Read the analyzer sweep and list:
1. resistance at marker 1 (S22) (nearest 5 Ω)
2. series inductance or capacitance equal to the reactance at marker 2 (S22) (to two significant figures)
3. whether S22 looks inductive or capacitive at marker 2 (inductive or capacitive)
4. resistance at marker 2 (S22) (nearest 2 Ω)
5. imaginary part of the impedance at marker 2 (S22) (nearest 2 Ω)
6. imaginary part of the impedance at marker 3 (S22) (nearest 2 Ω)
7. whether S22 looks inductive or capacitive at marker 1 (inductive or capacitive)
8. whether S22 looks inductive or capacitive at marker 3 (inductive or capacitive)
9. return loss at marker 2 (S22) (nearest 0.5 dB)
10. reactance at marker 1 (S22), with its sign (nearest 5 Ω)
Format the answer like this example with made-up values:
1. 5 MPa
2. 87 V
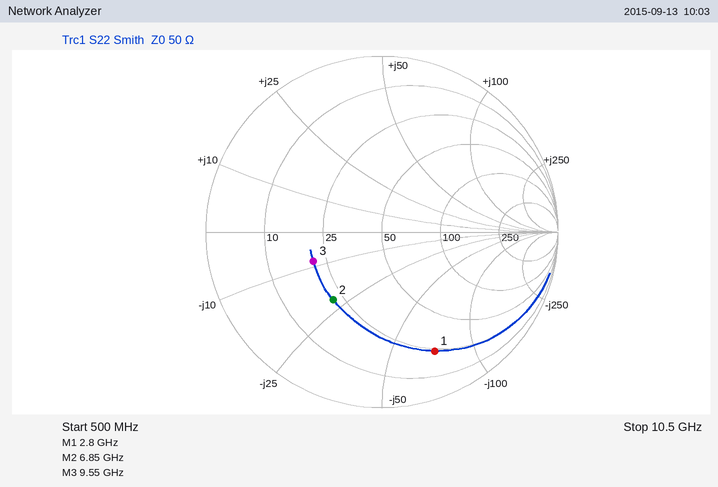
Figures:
1. 25 Ω
2. 1.1 pF
3. capacitive
4. 22 Ω
5. -22 Ω
6. -8 Ω
7. capacitive
8. capacitive
9. 6.5 dB
10. -70 Ω
